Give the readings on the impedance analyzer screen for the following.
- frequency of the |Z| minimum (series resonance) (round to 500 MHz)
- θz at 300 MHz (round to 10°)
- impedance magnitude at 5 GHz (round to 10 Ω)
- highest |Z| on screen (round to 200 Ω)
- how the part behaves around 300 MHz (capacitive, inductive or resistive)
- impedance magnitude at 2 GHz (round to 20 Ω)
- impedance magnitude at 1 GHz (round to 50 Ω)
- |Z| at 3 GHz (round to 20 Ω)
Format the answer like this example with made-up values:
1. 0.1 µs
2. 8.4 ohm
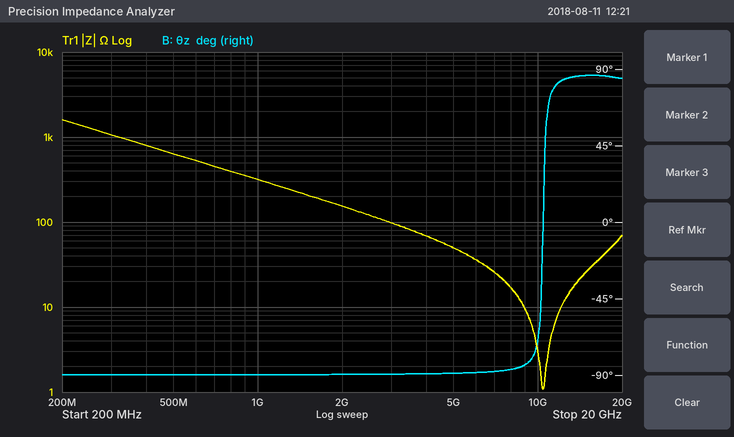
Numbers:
1. 10.5 GHz
2. -90°
3. 50 Ω
4. 1.6 kΩ
5. capacitive
6. 160 Ω
7. 300 Ω
8. 100 Ω
